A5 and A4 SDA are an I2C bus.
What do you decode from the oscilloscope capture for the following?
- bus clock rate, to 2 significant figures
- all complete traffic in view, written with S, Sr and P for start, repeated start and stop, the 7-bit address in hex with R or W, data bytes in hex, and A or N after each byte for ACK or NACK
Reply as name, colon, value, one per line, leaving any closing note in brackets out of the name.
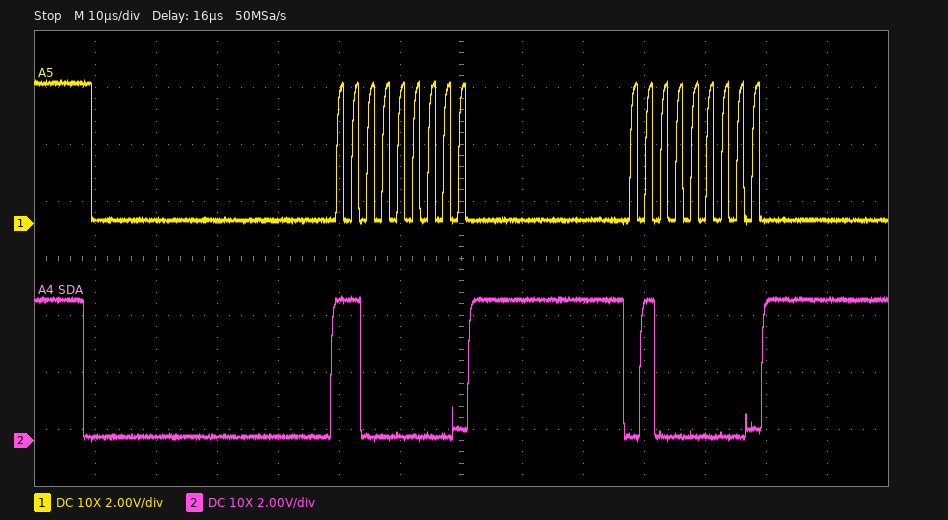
bus clock rate, to 2 significant figures: 400 kHz
all complete traffic in view, written with S, Sr and P for start, repeated start and stop, the 7-bit address in hex with R or W, data bytes in hex, and A or N after each byte for ACK or NACK: S 60W A 40 A
